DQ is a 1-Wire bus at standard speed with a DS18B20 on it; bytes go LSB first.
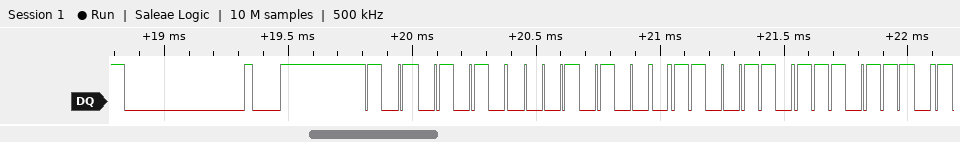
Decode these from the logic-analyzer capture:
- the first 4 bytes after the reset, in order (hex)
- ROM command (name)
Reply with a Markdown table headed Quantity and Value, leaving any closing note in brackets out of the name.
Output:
| Quantity | Value |
|---|---|
| the first 4 bytes after the reset, in order | 55 28 66 77 |
| ROM command | Match ROM |
